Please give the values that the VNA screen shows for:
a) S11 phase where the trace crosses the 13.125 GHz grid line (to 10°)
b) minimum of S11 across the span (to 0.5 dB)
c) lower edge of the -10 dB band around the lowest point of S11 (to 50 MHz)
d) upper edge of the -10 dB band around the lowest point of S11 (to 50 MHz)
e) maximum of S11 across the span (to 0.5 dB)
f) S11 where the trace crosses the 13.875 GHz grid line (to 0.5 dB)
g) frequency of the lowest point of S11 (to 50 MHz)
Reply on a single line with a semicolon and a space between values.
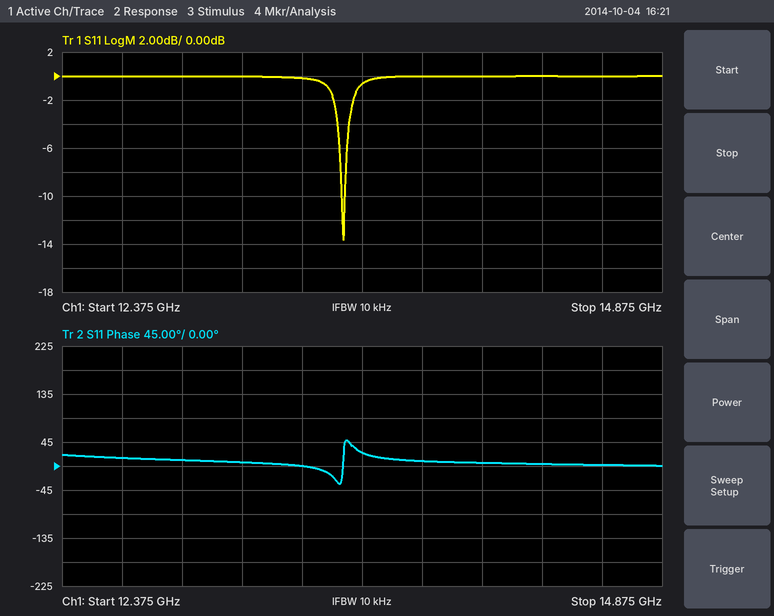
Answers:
10°; -13.5 dB; 13.55 GHz; 13.55 GHz; 0.0 dB; 0.0 dB; 13.55 GHz
